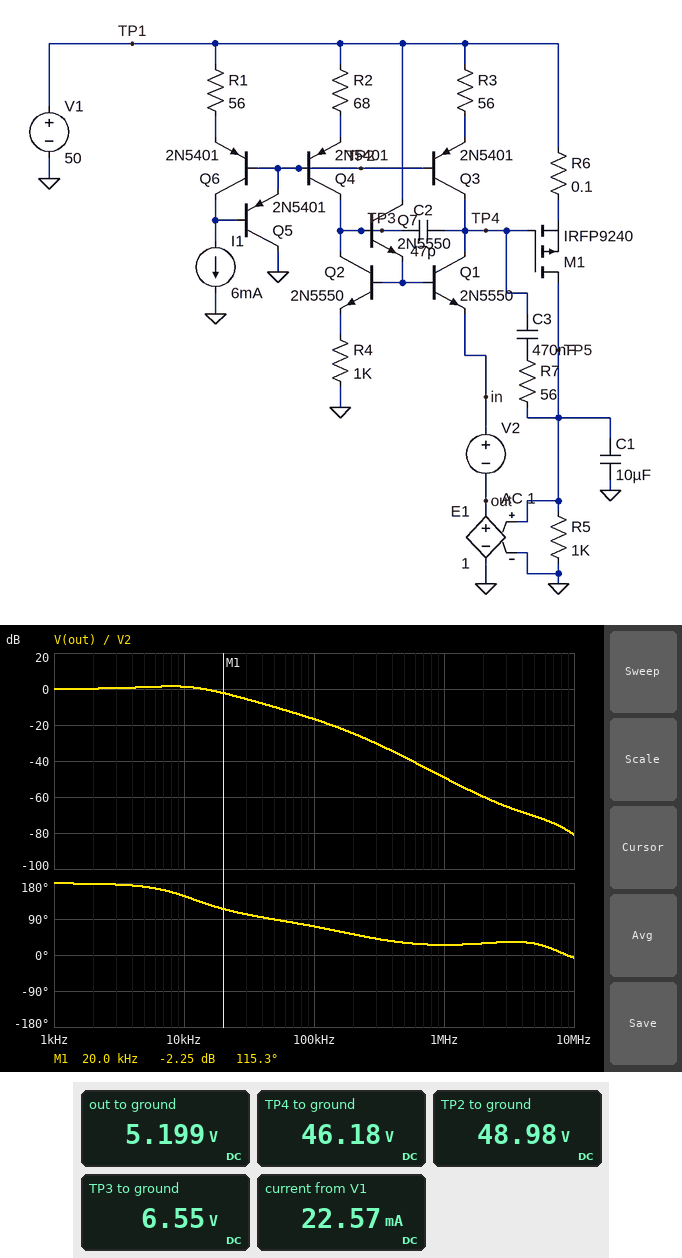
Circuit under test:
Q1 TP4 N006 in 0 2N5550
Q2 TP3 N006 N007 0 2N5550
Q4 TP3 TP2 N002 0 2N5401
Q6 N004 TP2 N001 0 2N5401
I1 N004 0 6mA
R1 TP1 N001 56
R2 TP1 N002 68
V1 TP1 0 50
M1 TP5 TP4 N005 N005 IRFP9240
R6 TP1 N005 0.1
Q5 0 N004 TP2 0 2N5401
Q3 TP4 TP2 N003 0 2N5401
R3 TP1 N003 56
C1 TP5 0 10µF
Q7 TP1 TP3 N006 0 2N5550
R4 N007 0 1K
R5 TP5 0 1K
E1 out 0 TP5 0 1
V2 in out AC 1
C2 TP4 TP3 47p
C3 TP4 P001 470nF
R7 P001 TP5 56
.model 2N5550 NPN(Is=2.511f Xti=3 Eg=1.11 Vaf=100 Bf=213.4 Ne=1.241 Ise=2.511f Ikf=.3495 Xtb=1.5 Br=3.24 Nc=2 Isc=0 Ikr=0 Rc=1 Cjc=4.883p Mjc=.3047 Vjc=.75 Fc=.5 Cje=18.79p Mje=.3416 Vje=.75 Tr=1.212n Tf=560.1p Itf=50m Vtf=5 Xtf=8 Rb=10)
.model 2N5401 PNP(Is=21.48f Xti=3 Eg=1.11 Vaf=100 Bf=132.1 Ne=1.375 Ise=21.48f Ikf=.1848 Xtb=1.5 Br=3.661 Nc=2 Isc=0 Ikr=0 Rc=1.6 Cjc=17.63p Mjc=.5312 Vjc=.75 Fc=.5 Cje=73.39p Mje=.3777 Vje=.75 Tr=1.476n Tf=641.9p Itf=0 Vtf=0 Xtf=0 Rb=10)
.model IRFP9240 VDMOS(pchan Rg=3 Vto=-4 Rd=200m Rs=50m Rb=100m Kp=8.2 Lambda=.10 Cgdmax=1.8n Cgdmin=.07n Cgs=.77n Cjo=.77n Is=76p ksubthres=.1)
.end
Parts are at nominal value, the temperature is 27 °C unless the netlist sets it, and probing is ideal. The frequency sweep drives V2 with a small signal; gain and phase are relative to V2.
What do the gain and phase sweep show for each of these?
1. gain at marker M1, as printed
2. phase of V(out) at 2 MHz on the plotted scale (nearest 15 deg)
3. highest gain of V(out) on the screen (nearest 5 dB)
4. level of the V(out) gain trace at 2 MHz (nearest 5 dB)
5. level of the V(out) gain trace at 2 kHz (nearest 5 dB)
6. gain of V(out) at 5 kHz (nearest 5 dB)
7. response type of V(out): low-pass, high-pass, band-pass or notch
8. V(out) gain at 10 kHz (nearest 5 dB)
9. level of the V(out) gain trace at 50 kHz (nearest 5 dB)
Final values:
-2.25 dB
30 deg
0 dB
-60 dB
0 dB
0 dB
low-pass
0 dB
-10 dB
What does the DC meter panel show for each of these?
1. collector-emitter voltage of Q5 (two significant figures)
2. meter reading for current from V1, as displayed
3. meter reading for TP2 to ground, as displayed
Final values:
-49 V
22.57 mA
48.98 V
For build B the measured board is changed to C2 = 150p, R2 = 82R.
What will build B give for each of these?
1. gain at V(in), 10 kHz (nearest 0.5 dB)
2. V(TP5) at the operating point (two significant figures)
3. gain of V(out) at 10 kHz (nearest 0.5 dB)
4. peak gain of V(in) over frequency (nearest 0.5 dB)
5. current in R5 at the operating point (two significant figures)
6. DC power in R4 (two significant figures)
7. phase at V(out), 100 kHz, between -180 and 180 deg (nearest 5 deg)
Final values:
-1.5 dB
4.4 V
2.0 dB
1.5 dB
4.4 mA
19 mW
40 deg
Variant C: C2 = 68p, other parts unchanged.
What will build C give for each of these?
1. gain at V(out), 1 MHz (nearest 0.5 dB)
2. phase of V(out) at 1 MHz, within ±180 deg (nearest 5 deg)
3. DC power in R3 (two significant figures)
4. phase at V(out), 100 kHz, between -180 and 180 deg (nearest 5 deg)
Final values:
-51.5 dB
30 deg
2.1 mW
65 deg
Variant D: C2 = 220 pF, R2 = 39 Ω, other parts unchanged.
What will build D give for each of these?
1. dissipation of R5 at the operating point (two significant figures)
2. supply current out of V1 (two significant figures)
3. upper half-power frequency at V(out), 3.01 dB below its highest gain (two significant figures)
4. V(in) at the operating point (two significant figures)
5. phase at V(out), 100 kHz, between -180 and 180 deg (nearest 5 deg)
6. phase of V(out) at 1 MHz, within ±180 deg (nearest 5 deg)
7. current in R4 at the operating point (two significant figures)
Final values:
76 mW
30 mA
33 kHz
8.7 V
40 deg
55 deg
8.7 mA
